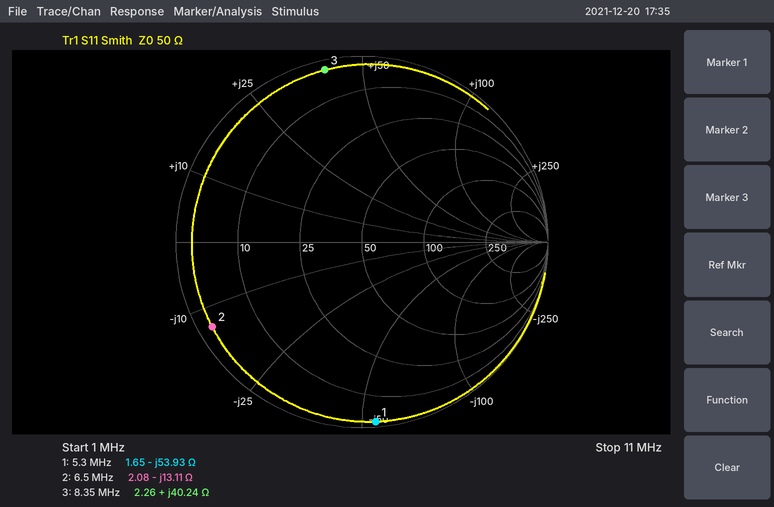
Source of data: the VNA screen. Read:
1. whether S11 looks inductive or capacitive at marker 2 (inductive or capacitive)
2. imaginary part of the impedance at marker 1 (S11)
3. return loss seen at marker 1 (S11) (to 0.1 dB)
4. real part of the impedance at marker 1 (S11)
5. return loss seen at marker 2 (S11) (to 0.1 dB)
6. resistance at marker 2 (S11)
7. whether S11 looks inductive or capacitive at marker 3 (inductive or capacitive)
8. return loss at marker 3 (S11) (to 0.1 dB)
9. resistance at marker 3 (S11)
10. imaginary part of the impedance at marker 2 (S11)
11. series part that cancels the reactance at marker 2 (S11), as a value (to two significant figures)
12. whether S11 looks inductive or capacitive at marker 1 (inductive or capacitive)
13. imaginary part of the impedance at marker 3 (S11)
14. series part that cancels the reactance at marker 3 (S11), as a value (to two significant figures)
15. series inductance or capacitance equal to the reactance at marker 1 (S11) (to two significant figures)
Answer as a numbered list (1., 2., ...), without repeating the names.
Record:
1. capacitive
2. -53.93 Ω
3. 0.3 dB
4. 1.65 Ω
5. 0.7 dB
6. 2.08 Ω
7. inductive
8. 0.5 dB
9. 2.26 Ω
10. -13.11 Ω
11. 320 nH
12. capacitive
13. +40.24 Ω
14. 470 pF
15. 560 pF
